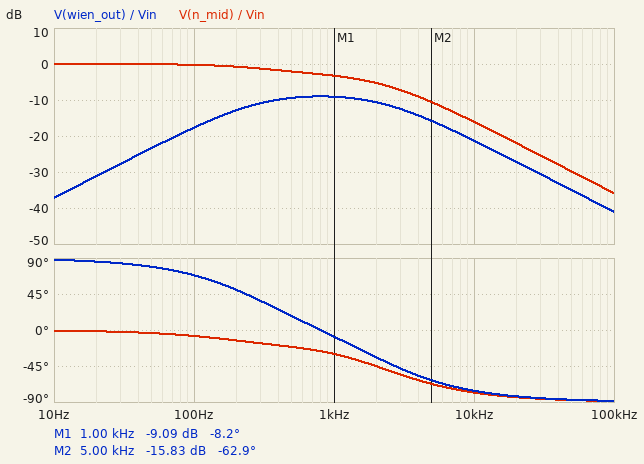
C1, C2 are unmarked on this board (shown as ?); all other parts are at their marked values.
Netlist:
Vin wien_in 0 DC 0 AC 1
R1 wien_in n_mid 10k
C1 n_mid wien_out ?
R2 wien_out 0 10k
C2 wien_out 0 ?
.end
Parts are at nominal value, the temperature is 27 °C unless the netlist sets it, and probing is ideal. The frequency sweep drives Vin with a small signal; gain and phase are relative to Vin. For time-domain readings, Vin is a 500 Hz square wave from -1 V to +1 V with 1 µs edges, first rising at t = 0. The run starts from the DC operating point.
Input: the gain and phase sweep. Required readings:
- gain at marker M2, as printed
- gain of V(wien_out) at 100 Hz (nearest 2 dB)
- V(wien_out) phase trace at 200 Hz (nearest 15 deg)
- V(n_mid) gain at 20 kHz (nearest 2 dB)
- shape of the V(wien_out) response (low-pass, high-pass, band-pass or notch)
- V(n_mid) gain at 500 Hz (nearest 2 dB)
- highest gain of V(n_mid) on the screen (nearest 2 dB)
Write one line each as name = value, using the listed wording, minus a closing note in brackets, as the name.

gain at marker M2, as printed = -15.83 dB
gain of V(wien_out) at 100 Hz = -18 dB
V(wien_out) phase trace at 200 Hz = 45 deg
V(n_mid) gain at 20 kHz = -22 dB
shape of the V(wien_out) response = band-pass
V(n_mid) gain at 500 Hz = -2 dB
highest gain of V(n_mid) on the screen = 0 dB
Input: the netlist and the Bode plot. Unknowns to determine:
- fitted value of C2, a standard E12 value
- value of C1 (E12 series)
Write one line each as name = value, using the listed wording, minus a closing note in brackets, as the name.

fitted value of C2, a standard E12 value = 18 nF
value of C1 = 22 nF
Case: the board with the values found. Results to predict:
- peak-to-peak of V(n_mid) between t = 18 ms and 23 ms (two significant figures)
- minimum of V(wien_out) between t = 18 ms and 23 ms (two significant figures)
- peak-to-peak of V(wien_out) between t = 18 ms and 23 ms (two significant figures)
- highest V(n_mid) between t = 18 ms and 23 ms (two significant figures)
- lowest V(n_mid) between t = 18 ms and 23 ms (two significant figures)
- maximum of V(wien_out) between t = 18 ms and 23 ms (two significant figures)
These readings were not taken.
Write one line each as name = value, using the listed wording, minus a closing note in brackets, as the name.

peak-to-peak of V(n_mid) between t = 18 ms and 23 ms = 1.8 V
minimum of V(wien_out) between t = 18 ms and 23 ms = -500 mV
peak-to-peak of V(wien_out) between t = 18 ms and 23 ms = 990 mV
highest V(n_mid) between t = 18 ms and 23 ms = 910 mV
lowest V(n_mid) between t = 18 ms and 23 ms = -910 mV
maximum of V(wien_out) between t = 18 ms and 23 ms = 500 mV
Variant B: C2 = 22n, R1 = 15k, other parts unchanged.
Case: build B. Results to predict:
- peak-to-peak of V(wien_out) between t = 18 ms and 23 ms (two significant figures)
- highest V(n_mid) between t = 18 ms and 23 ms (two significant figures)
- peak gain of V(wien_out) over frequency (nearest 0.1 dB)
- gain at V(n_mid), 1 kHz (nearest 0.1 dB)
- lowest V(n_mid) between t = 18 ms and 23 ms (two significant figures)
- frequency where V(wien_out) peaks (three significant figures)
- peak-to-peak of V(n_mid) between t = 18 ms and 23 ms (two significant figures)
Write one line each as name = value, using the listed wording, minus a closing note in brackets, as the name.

peak-to-peak of V(wien_out) between t = 18 ms and 23 ms = 730 mV
highest V(n_mid) between t = 18 ms and 23 ms = 860 mV
peak gain of V(wien_out) over frequency = -10.9 dB
gain at V(n_mid), 1 kHz = -4.9 dB
lowest V(n_mid) between t = 18 ms and 23 ms = -860 mV
frequency where V(wien_out) peaks = 591 Hz
peak-to-peak of V(n_mid) between t = 18 ms and 23 ms = 1.7 V
